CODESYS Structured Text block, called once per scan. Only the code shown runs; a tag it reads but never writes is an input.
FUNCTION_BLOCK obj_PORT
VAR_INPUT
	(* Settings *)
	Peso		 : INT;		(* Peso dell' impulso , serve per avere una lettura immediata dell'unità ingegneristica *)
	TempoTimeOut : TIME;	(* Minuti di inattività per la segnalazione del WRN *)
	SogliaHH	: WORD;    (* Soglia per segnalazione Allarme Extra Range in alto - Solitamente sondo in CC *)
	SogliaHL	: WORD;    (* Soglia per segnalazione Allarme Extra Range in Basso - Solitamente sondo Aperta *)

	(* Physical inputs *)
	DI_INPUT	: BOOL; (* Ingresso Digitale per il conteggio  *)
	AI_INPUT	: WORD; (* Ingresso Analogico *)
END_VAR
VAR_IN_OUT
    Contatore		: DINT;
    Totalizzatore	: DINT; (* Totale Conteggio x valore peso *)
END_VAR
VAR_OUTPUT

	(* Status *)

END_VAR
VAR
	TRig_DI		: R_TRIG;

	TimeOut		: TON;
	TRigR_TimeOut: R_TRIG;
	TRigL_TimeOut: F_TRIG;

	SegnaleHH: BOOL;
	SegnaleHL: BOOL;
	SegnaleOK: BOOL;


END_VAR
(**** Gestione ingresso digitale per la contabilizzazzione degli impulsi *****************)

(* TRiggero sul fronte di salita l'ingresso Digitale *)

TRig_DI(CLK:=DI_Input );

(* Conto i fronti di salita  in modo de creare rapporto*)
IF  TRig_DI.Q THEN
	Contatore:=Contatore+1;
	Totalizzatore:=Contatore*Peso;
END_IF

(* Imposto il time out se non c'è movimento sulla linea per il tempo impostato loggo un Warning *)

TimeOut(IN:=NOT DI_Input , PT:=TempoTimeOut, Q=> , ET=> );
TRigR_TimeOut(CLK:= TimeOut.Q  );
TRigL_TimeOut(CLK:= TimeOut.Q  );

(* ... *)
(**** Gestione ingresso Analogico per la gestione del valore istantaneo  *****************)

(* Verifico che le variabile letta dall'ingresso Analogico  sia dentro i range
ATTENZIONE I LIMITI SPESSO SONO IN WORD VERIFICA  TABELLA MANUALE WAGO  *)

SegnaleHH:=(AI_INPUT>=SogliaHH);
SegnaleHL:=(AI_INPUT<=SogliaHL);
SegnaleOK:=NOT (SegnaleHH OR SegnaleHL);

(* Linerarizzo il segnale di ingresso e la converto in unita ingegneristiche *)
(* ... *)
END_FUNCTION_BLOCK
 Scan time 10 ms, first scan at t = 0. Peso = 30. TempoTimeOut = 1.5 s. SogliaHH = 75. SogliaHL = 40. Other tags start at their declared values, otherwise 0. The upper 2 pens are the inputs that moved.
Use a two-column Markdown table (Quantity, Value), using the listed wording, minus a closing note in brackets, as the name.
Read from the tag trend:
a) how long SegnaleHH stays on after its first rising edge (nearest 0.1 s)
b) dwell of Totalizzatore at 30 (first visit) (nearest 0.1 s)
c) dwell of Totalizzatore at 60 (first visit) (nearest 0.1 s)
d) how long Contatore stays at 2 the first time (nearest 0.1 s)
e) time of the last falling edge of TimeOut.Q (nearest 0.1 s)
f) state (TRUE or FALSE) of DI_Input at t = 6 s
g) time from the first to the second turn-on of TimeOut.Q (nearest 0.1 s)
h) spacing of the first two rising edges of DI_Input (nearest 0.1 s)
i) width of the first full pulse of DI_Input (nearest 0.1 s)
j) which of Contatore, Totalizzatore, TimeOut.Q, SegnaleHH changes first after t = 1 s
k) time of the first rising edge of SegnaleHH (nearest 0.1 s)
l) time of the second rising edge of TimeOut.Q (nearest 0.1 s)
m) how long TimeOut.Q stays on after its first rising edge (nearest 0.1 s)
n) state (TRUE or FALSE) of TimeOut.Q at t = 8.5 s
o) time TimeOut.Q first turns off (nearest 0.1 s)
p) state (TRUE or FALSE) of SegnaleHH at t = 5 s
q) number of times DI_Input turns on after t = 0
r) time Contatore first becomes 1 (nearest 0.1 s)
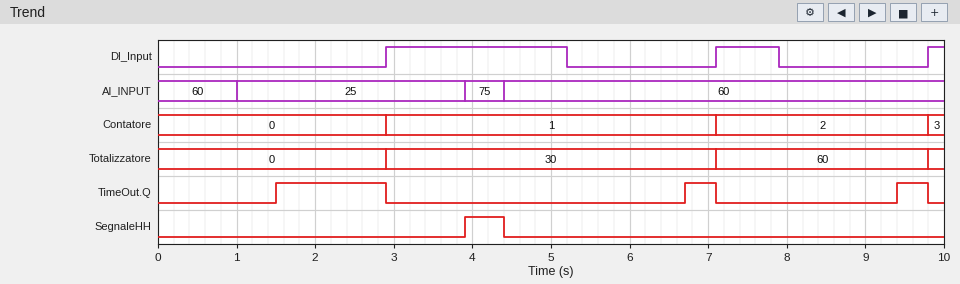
| Quantity | Value |
|---|---|
| how long SegnaleHH stays on after its first rising edge | 0.5 s |
| dwell of Totalizzatore at 30 (first visit) | 4.2 s |
| dwell of Totalizzatore at 60 (first visit) | 2.7 s |
| how long Contatore stays at 2 the first time | 2.7 s |
| time of the last falling edge of TimeOut.Q | 9.8 s |
| state (TRUE or FALSE) of DI_Input at t = 6 s | FALSE |
| time from the first to the second turn-on of TimeOut.Q | 5.2 s |
| spacing of the first two rising edges of DI_Input | 4.2 s |
| width of the first full pulse of DI_Input | 2.3 s |
| which of Contatore, Totalizzatore, TimeOut.Q, SegnaleHH changes first after t = 1 s | TimeOut.Q |
| time of the first rising edge of SegnaleHH | 3.9 s |
| time of the second rising edge of TimeOut.Q | 6.7 s |
| how long TimeOut.Q stays on after its first rising edge | 1.4 s |
| state (TRUE or FALSE) of TimeOut.Q at t = 8.5 s | FALSE |
| time TimeOut.Q first turns off | 2.9 s |
| state (TRUE or FALSE) of SegnaleHH at t = 5 s | FALSE |
| number of times DI_Input turns on after t = 0 | 3 |
| time Contatore first becomes 1 | 2.9 s |
